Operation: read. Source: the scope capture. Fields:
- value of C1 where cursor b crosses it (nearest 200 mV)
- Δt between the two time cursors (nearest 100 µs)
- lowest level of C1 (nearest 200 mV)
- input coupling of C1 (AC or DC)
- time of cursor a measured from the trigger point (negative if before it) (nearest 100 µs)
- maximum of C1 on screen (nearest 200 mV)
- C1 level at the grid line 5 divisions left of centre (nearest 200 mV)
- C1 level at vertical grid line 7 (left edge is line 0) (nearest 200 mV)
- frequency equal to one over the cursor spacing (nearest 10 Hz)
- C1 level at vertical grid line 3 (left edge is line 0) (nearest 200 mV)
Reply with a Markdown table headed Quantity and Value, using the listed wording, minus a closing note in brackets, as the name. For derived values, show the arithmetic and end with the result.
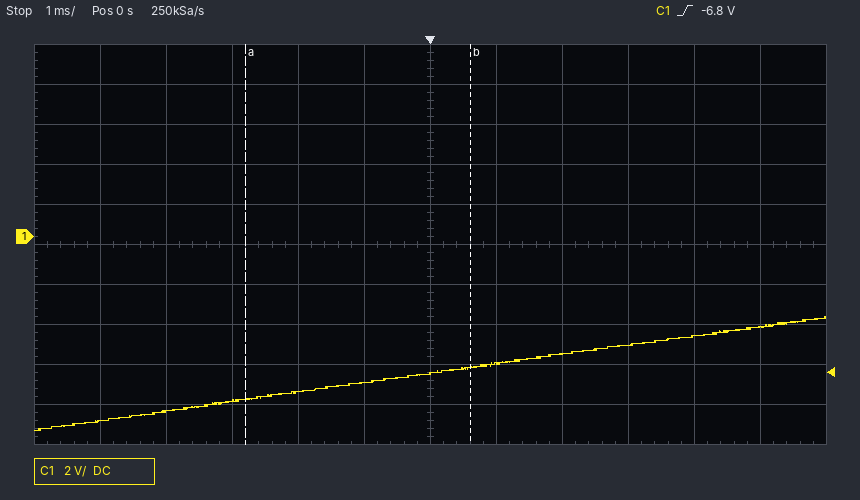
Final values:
| Quantity | Value |
|---|---|
| value of C1 where cursor b crosses it | -6.6 V |
| Δt between the two time cursors | 3.4 ms |
| lowest level of C1 | -9.6 V |
| input coupling of C1 | DC |
| time of cursor a measured from the trigger point (negative if before it) | -2.8 ms |
| maximum of C1 on screen | -4.0 V |
| C1 level at the grid line 5 divisions left of centre | -9.2 V |
| C1 level at vertical grid line 7 (left edge is line 0) | -6.4 V |
| frequency equal to one over the cursor spacing | 1 / 3.4 ms ≈ 290 Hz |
| C1 level at vertical grid line 3 (left edge is line 0) | -8.2 V |
